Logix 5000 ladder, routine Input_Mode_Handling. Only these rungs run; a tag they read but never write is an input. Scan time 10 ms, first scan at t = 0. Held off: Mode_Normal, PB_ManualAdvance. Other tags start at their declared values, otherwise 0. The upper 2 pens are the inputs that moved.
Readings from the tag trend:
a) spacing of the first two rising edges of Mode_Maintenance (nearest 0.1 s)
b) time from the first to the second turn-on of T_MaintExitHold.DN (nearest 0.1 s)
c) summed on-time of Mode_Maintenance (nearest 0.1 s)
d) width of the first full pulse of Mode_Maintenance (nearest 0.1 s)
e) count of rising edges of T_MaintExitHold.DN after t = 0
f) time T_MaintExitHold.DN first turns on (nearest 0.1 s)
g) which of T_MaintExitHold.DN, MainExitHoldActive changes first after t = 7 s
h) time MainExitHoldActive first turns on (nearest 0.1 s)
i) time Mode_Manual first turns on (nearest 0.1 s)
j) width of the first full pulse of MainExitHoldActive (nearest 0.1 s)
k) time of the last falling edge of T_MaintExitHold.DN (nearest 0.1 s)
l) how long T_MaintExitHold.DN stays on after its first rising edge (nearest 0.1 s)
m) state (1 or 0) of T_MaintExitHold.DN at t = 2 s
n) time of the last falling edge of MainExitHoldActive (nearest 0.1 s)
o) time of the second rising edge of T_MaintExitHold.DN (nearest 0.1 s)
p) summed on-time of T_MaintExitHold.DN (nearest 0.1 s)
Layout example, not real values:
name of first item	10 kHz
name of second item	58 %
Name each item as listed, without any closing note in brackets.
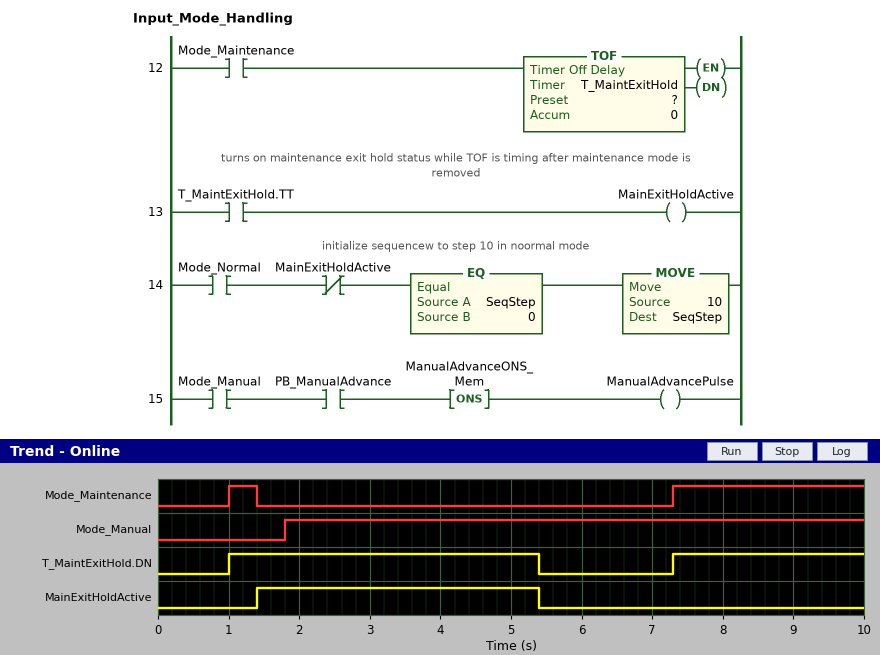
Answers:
spacing of the first two rising edges of Mode_Maintenance	6.3 s
time from the first to the second turn-on of T_MaintExitHold.DN	6.3 s
summed on-time of Mode_Maintenance	3.1 s
width of the first full pulse of Mode_Maintenance	0.4 s
count of rising edges of T_MaintExitHold.DN after t = 0	2
time T_MaintExitHold.DN first turns on	1.0 s
which of T_MaintExitHold.DN, MainExitHoldActive changes first after t = 7 s	T_MaintExitHold.DN
time MainExitHoldActive first turns on	1.4 s
time Mode_Manual first turns on	1.8 s
width of the first full pulse of MainExitHoldActive	4.0 s
time of the last falling edge of T_MaintExitHold.DN	5.4 s
how long T_MaintExitHold.DN stays on after its first rising edge	4.4 s
state (1 or 0) of T_MaintExitHold.DN at t = 2 s	1
time of the last falling edge of MainExitHoldActive	5.4 s
time of the second rising edge of T_MaintExitHold.DN	7.3 s
summed on-time of T_MaintExitHold.DN	7.1 s
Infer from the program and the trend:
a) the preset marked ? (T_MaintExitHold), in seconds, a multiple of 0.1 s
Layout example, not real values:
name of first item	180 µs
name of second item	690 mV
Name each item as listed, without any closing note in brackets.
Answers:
the preset marked ? (T_MaintExitHold), in seconds, a multiple of 0.1 s	4.0 s
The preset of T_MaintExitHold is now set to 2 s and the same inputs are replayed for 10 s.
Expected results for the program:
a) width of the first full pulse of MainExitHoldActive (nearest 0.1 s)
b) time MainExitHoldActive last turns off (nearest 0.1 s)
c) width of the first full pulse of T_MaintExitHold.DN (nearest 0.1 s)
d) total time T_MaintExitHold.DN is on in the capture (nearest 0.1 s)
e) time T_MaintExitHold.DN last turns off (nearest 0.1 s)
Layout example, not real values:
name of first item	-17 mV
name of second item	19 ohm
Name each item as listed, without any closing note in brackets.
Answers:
width of the first full pulse of MainExitHoldActive	2.0 s
time MainExitHoldActive last turns off	3.4 s
width of the first full pulse of T_MaintExitHold.DN	2.4 s
total time T_MaintExitHold.DN is on in the capture	5.1 s
time T_MaintExitHold.DN last turns off	3.4 s
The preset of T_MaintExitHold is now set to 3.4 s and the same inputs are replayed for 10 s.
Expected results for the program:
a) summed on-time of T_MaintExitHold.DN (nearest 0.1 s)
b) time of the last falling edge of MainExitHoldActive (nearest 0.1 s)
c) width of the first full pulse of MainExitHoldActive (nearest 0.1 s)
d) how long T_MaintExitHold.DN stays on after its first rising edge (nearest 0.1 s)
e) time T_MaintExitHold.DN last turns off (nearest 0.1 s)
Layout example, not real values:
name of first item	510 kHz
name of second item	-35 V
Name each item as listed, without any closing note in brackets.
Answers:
summed on-time of T_MaintExitHold.DN	6.5 s
time of the last falling edge of MainExitHoldActive	4.8 s
width of the first full pulse of MainExitHoldActive	3.4 s
how long T_MaintExitHold.DN stays on after its first rising edge	3.8 s
time T_MaintExitHold.DN last turns off	4.8 s
